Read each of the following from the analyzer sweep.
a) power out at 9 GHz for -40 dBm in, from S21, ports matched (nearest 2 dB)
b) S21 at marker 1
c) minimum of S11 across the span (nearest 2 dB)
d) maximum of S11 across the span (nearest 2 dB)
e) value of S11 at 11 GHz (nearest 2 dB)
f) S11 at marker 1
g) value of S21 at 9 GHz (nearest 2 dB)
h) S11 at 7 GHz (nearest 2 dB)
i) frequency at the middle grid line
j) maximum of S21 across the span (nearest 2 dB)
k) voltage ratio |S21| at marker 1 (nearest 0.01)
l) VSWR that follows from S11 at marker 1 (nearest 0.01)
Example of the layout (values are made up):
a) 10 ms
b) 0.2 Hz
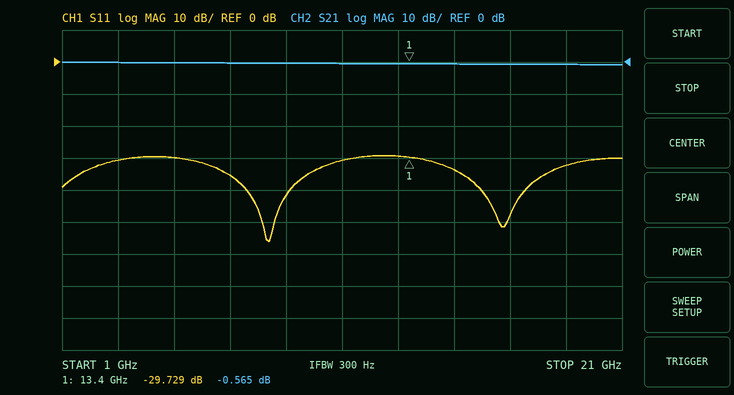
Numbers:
a) -40 dBm
b) -0.565 dB
c) -56 dB
d) -30 dB
e) -30 dB
f) -29.729 dB
g) 0 dB
h) -36 dB
i) 11 GHz
j) 0 dB
k) 0.94
l) 1.07
